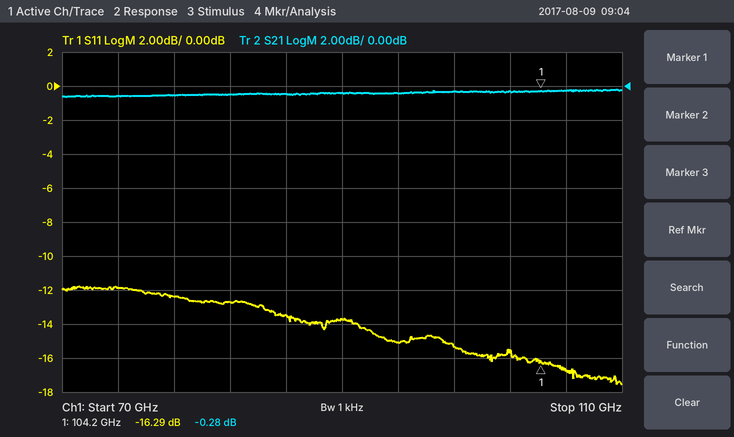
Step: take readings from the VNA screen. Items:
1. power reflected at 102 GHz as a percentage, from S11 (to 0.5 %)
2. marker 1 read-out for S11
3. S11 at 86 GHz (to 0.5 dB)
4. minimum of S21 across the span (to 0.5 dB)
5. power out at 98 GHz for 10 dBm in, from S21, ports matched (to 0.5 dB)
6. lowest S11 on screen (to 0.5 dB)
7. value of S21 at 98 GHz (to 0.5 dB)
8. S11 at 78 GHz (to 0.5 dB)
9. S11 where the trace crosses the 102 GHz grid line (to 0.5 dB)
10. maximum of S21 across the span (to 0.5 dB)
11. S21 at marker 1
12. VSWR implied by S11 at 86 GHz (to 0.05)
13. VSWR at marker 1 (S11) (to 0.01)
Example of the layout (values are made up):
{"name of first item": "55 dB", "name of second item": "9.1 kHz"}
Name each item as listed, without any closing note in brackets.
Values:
{"power reflected at 102 GHz as a percentage, from S11": "3.0 %", "marker 1 read-out for S11": "-16.29 dB", "S11 at 86 GHz": "-13.5 dB", "minimum of S21 across the span": "-0.5 dB", "power out at 98 GHz for 10 dBm in, from S21, ports matched": "9.5 dBm", "lowest S11 on screen": "-17.5 dB", "value of S21 at 98 GHz": "-0.5 dB", "S11 at 78 GHz": "-12.5 dB", "S11 where the trace crosses the 102 GHz grid line": "-15.5 dB", "maximum of S21 across the span": "0.0 dB", "S21 at marker 1": "-0.28 dB", "VSWR implied by S11 at 86 GHz": "1.55", "VSWR at marker 1 (S11)": "1.36"}
